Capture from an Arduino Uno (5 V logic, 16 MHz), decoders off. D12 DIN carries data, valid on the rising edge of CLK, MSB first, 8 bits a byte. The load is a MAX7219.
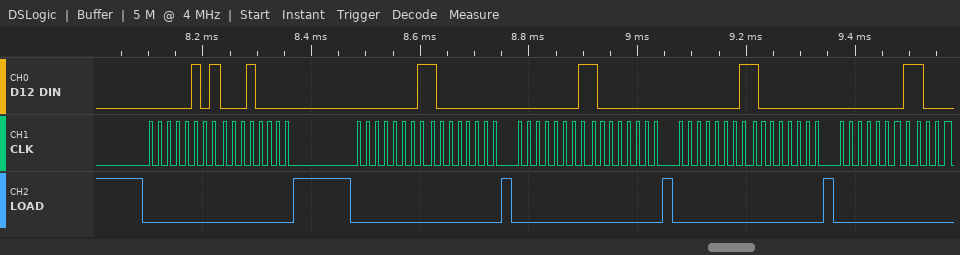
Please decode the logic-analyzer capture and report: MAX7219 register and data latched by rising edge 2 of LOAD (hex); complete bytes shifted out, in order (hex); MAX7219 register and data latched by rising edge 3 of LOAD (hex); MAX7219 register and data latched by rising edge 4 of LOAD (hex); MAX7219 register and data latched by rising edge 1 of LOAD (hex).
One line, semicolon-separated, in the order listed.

register 0x1, data 0x80; 0x05 0x10 0x01 0x80 0x01 0x80 0x01 0x80 0x01; register 0x1, data 0x80; register 0x1, data 0x80; register 0x5, data 0x10
